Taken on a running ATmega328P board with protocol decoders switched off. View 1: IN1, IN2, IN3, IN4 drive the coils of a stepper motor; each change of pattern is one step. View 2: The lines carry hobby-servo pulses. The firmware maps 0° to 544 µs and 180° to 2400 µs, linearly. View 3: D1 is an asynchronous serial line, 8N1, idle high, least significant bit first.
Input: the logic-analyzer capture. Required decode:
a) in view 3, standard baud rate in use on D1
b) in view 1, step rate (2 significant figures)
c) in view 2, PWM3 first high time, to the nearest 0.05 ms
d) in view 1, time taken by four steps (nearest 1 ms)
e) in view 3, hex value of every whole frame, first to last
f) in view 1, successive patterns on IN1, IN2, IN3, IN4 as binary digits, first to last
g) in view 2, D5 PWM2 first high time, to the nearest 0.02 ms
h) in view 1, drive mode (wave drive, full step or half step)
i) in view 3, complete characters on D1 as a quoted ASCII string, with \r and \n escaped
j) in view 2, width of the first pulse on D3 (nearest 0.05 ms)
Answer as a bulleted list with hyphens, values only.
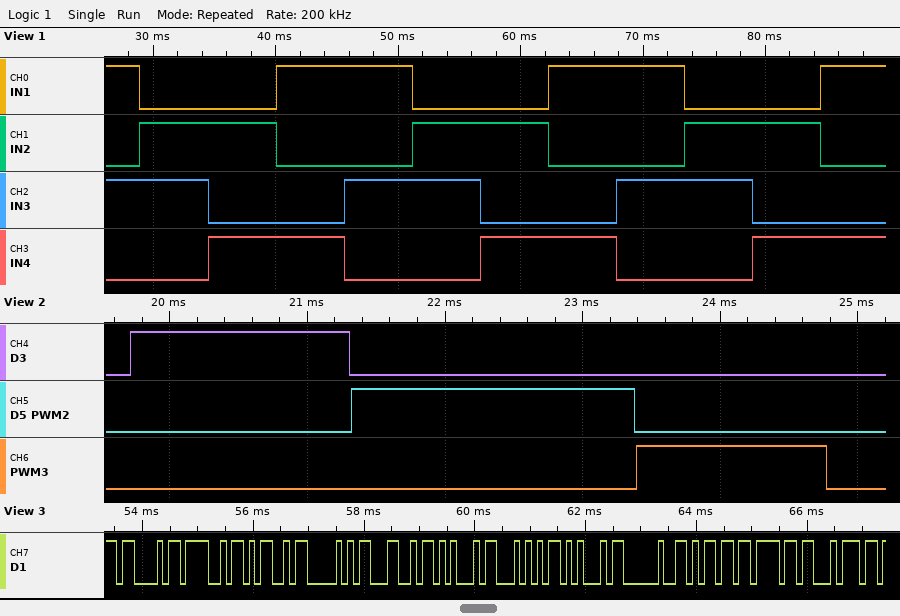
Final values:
- 9600 baud
- 180 steps/s
- 1.40 ms
- 22 ms
- 43 4F 4D 50 4C 45 54 45 20 6D 6F 74
- 1010 0110 0101 1001 1010 0110 0101 1001 1010 0110 0101 1001
- 2.06 ms
- full step
- "COMPLETE mot"
- 1.60 ms
